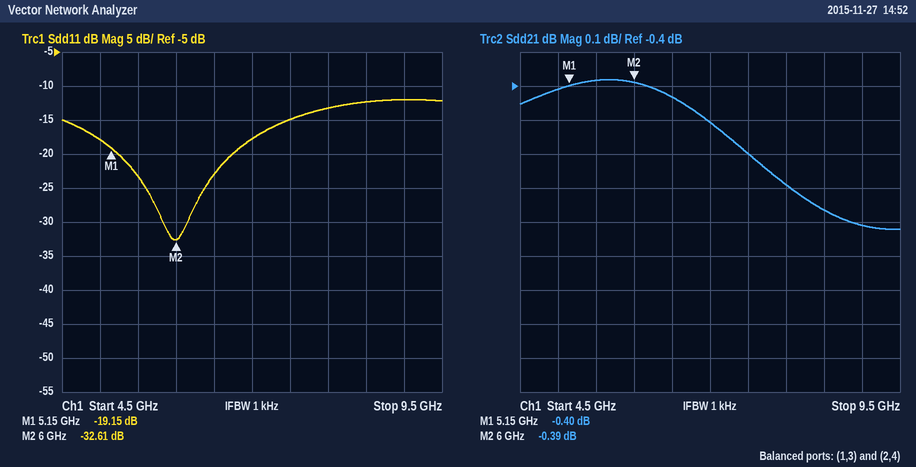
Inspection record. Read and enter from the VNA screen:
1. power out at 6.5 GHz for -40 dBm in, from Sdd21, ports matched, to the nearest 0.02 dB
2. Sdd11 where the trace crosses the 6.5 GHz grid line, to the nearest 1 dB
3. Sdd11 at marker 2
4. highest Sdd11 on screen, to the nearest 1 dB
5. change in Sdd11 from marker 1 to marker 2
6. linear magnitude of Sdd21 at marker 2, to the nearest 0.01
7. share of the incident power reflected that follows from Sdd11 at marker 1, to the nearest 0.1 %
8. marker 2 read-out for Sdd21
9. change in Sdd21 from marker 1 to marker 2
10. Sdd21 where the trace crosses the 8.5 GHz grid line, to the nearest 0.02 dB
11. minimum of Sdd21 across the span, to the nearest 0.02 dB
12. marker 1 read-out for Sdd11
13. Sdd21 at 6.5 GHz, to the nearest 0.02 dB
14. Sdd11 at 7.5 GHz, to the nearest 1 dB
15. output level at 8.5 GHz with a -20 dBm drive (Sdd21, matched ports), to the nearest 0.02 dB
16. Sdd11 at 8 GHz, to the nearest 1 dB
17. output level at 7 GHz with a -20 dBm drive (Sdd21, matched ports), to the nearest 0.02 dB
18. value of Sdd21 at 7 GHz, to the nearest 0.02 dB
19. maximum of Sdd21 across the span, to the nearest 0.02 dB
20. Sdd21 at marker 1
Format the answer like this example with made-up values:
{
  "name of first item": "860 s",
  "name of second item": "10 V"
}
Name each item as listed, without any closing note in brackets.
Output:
{
  "power out at 6.5 GHz for -40 dBm in, from Sdd21, ports matched, to the nearest 0.02 dB": "-40.44 dBm",
  "Sdd11 where the trace crosses the 6.5 GHz grid line, to the nearest 1 dB": "-23 dB",
  "Sdd11 at marker 2": "-32.61 dB",
  "highest Sdd11 on screen, to the nearest 1 dB": "-12 dB",
  "change in Sdd11 from marker 1 to marker 2": "-13.46 dB",
  "linear magnitude of Sdd21 at marker 2, to the nearest 0.01": "0.96",
  "share of the incident power reflected that follows from Sdd11 at marker 1, to the nearest 0.1 %": "1.2 %",
  "marker 2 read-out for Sdd21": "-0.39 dB",
  "change in Sdd21 from marker 1 to marker 2": "0.01 dB",
  "Sdd21 where the trace crosses the 8.5 GHz grid line, to the nearest 0.02 dB": "-0.76 dB",
  "minimum of Sdd21 across the span, to the nearest 0.02 dB": "-0.82 dB",
  "marker 1 read-out for Sdd11": "-19.15 dB",
  "Sdd21 at 6.5 GHz, to the nearest 0.02 dB": "-0.44 dB",
  "Sdd11 at 7.5 GHz, to the nearest 1 dB": "-15 dB",
  "output level at 8.5 GHz with a -20 dBm drive (Sdd21, matched ports), to the nearest 0.02 dB": "-20.76 dBm",
  "Sdd11 at 8 GHz, to the nearest 1 dB": "-13 dB",
  "output level at 7 GHz with a -20 dBm drive (Sdd21, matched ports), to the nearest 0.02 dB": "-20.50 dBm",
  "value of Sdd21 at 7 GHz, to the nearest 0.02 dB": "-0.50 dB",
  "maximum of Sdd21 across the span, to the nearest 0.02 dB": "-0.38 dB",
  "Sdd21 at marker 1": "-0.40 dB"
}
